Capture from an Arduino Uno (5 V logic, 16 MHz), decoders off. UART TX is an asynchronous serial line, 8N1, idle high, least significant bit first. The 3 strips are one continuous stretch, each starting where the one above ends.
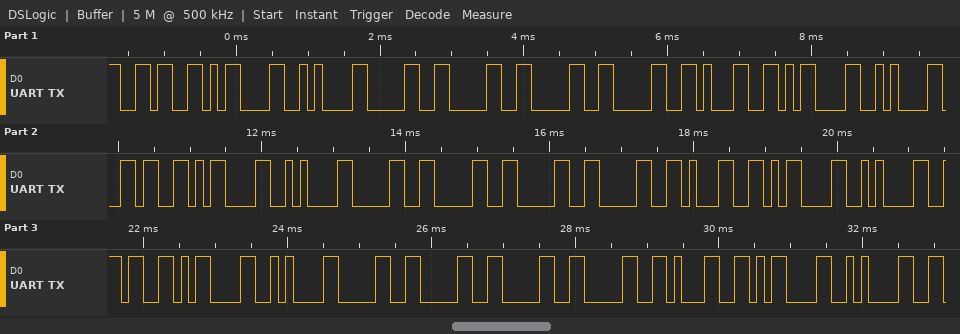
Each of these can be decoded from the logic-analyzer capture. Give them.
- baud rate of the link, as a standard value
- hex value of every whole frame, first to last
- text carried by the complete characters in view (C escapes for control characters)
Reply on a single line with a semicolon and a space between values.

9600 baud; 36 0D 0A 30 30 30 30 31 0D 0A 36 0D 0A 30 30 30 30 31 0D 0A 36 0D 0A 30 30 30 30 31 0D 0A; "6\r\n00001\r\n6\r\n00001\r\n6\r\n00001\r\n"
